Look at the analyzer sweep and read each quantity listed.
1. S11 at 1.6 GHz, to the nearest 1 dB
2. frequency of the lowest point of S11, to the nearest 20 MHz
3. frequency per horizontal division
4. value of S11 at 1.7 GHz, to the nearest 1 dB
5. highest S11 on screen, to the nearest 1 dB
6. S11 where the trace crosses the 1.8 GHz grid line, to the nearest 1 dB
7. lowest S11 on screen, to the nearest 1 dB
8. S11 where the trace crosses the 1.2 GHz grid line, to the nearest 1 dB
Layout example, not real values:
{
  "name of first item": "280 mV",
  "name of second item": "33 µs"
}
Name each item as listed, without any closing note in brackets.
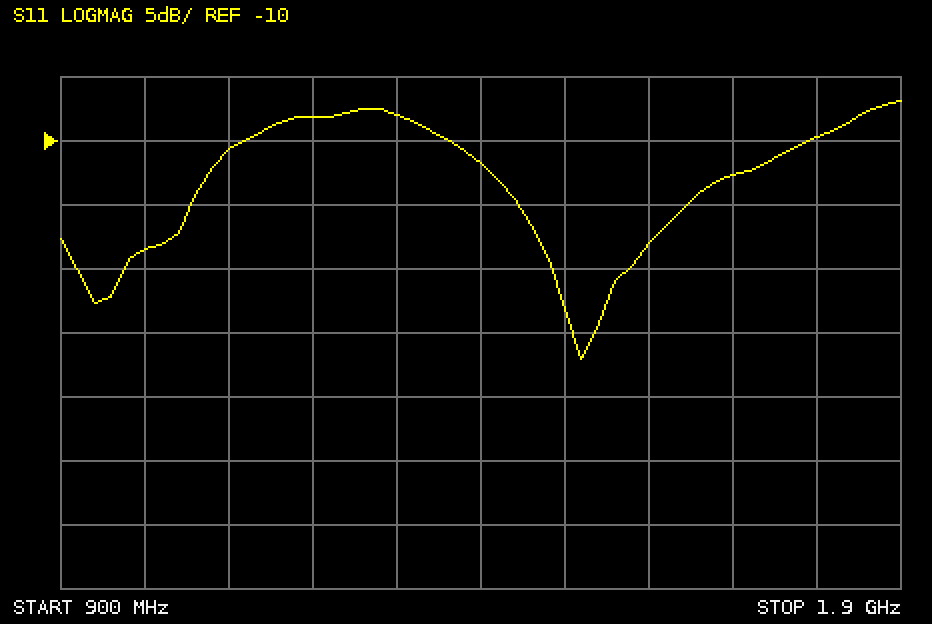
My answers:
{
  "S11 at 1.6 GHz, to the nearest 1 dB": "-18 dB",
  "frequency of the lowest point of S11, to the nearest 20 MHz": "1.52 GHz",
  "frequency per horizontal division": "100 MHz",
  "value of S11 at 1.7 GHz, to the nearest 1 dB": "-13 dB",
  "highest S11 on screen, to the nearest 1 dB": "-7 dB",
  "S11 where the trace crosses the 1.8 GHz grid line, to the nearest 1 dB": "-10 dB",
  "lowest S11 on screen, to the nearest 1 dB": "-27 dB",
  "S11 where the trace crosses the 1.2 GHz grid line, to the nearest 1 dB": "-8 dB"
}
